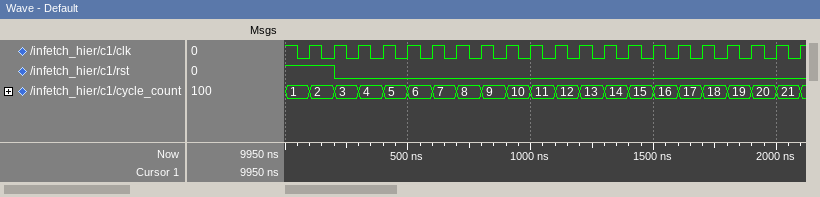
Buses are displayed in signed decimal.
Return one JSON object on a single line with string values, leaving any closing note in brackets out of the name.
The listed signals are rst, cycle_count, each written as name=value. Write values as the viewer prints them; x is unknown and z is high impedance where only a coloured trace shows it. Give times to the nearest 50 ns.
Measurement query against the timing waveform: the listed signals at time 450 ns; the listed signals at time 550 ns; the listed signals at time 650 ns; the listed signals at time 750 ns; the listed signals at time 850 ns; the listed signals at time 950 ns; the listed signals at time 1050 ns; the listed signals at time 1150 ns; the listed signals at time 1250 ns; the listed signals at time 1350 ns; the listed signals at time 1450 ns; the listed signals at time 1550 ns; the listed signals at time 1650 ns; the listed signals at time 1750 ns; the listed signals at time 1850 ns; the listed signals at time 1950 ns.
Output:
{"the listed signals at time 450 ns": "rst=0, cycle_count=5", "the listed signals at time 550 ns": "rst=0, cycle_count=6", "the listed signals at time 650 ns": "rst=0, cycle_count=7", "the listed signals at time 750 ns": "rst=0, cycle_count=8", "the listed signals at time 850 ns": "rst=0, cycle_count=9", "the listed signals at time 950 ns": "rst=0, cycle_count=10", "the listed signals at time 1050 ns": "rst=0, cycle_count=11", "the listed signals at time 1150 ns": "rst=0, cycle_count=12", "the listed signals at time 1250 ns": "rst=0, cycle_count=13", "the listed signals at time 1350 ns": "rst=0, cycle_count=14", "the listed signals at time 1450 ns": "rst=0, cycle_count=15", "the listed signals at time 1550 ns": "rst=0, cycle_count=16", "the listed signals at time 1650 ns": "rst=0, cycle_count=17", "the listed signals at time 1750 ns": "rst=0, cycle_count=18", "the listed signals at time 1850 ns": "rst=0, cycle_count=19", "the listed signals at time 1950 ns": "rst=0, cycle_count=20"}
